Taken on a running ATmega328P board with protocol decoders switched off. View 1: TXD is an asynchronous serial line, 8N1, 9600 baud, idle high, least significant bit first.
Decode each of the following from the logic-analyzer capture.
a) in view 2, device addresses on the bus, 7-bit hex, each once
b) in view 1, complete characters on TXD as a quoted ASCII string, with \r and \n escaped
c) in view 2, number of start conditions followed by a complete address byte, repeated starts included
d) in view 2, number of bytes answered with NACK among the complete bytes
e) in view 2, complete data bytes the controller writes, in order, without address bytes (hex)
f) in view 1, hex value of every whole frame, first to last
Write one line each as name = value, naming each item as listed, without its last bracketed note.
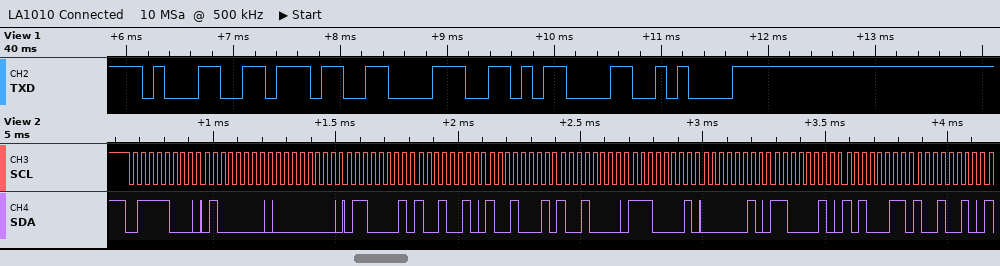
in view 2, device addresses on the bus, 7-bit hex, each once = 0x3C
in view 1, complete characters on TXD as a quoted ASCII string, with \r and \n escaped = "178\r\n"
in view 2, number of start conditions followed by a complete address byte, repeated starts included = 1
in view 2, number of bytes answered with NACK among the complete bytes = 0
in view 2, complete data bytes the controller writes, in order, without address bytes = 40 00 61 92 91 90 E1 02 C2 A3 92
in view 1, hex value of every whole frame, first to last = 31 37 38 0D 0A
